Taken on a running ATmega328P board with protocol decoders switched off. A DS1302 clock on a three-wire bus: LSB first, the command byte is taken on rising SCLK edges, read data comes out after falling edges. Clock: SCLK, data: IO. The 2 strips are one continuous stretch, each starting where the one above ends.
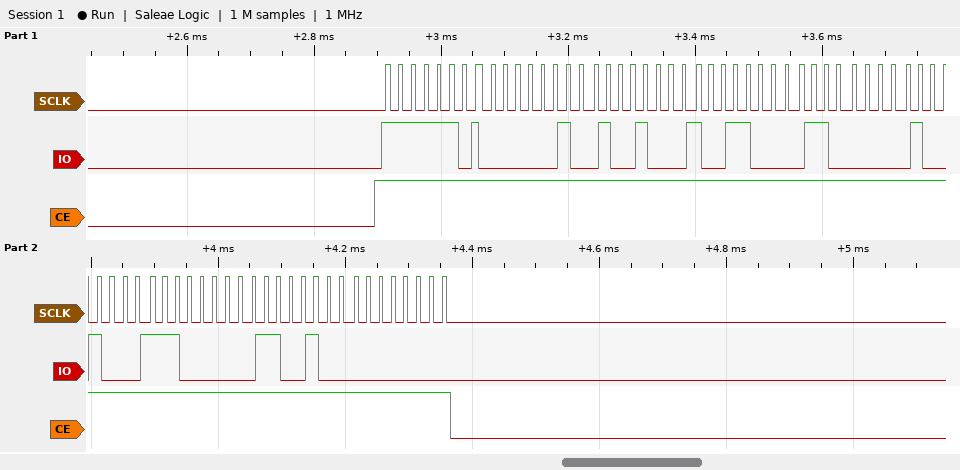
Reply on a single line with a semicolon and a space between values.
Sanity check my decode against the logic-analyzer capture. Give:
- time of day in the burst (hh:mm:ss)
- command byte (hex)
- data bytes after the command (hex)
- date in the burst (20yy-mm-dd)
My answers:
19:12:40; 0xBF; 40 12 19 06 12 07 26 00; 2026-12-06
